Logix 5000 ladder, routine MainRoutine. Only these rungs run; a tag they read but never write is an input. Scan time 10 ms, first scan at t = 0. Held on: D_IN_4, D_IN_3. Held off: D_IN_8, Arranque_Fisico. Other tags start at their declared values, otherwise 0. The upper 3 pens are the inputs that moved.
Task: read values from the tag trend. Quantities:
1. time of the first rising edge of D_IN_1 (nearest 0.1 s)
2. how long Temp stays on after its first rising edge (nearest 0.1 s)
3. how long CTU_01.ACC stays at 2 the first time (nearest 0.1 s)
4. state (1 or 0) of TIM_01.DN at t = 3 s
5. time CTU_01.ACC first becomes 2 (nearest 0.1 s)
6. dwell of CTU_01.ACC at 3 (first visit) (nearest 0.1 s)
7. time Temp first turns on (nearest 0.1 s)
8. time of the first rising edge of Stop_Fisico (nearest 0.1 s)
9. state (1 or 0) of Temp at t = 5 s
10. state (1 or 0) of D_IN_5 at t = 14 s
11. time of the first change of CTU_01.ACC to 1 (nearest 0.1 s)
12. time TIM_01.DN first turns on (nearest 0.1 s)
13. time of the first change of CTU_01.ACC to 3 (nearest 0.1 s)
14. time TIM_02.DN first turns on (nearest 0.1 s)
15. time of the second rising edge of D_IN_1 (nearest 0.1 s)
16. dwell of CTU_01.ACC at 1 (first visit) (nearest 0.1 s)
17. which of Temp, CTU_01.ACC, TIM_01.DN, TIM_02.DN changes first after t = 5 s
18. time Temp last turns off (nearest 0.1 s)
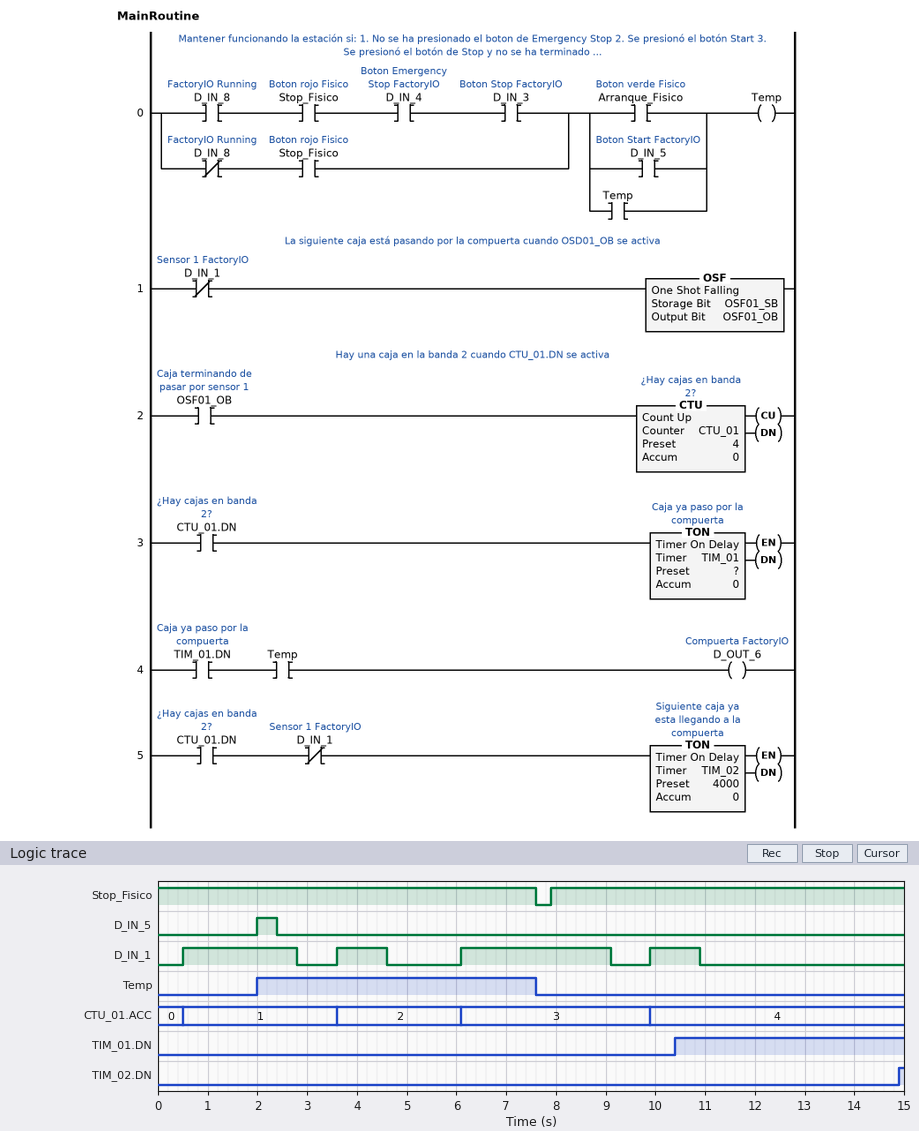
0.5 s
5.6 s
2.5 s
0
3.6 s
3.8 s
2.0 s
7.9 s
1
0
0.5 s
10.4 s
6.1 s
14.9 s
3.6 s
3.1 s
CTU_01.ACC
7.6 s
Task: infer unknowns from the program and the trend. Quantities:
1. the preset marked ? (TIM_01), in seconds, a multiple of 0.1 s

0.5 s
